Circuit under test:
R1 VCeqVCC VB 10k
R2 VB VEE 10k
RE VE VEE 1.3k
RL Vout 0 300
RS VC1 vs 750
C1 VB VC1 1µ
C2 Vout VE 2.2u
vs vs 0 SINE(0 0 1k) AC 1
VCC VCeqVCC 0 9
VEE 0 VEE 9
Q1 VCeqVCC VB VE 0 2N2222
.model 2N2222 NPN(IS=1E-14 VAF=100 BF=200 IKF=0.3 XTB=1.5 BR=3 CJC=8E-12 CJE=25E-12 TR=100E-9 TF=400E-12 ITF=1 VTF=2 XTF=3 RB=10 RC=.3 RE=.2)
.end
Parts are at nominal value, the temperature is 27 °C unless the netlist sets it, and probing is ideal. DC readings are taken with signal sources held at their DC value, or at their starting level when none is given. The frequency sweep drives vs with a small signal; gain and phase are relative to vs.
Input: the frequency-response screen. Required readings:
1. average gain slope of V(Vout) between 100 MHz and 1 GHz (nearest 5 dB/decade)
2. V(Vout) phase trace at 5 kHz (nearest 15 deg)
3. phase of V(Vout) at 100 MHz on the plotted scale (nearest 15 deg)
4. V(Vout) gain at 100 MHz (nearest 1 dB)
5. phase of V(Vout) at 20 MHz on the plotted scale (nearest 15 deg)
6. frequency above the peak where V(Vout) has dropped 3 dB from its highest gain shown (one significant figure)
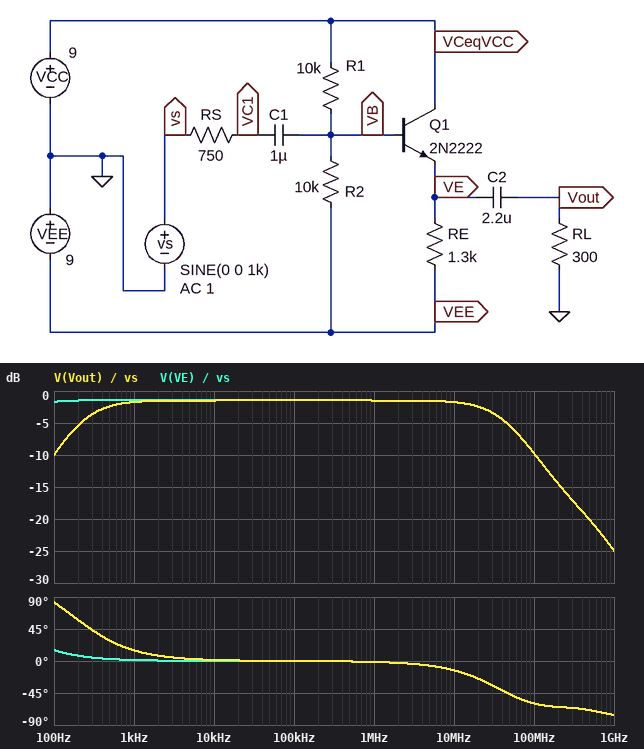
-15 dB/decade
0 deg
-60 deg
-10 dB
-30 deg
40 MHz
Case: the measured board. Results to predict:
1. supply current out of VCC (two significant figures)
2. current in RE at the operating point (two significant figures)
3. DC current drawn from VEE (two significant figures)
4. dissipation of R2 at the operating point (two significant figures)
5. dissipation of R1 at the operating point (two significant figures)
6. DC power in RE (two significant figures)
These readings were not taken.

7.2 mA
6.3 mA
7.2 mA
7.8 mW
8.4 mW
51 mW
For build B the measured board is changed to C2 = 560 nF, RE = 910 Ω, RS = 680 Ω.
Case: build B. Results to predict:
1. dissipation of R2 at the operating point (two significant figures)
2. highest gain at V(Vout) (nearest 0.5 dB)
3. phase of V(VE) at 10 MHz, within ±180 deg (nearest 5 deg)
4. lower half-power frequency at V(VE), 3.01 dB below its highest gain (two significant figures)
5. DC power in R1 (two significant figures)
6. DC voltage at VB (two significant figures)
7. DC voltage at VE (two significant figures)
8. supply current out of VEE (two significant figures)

7.7 mW
-1.5 dB
-10 deg
28 Hz
8.5 mW
-210 mV
-920 mV
9.8 mA
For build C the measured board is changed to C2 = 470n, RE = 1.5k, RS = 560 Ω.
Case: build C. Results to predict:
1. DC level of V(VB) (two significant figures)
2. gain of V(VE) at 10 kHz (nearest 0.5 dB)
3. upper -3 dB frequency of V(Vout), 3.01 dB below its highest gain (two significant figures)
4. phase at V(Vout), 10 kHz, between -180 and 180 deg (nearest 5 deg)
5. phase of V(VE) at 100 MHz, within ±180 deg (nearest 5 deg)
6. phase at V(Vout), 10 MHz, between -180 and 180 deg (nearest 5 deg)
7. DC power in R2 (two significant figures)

-130 mV
-1.0 dB
51 MHz
5 deg
-55 deg
-10 deg
7.9 mW
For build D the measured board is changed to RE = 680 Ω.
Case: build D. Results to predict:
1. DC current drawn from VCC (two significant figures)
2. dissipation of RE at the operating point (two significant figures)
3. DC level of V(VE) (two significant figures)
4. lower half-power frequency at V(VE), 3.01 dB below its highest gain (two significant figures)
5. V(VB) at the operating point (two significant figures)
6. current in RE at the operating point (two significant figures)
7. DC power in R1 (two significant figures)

13 mA
94 mW
-1.0 V
28 Hz
-280 mV
12 mA
8.6 mW
